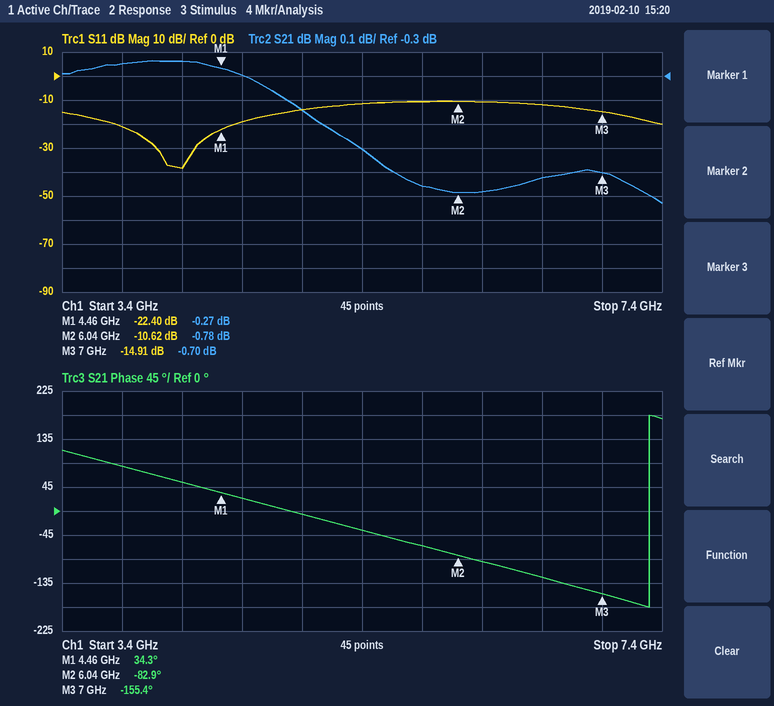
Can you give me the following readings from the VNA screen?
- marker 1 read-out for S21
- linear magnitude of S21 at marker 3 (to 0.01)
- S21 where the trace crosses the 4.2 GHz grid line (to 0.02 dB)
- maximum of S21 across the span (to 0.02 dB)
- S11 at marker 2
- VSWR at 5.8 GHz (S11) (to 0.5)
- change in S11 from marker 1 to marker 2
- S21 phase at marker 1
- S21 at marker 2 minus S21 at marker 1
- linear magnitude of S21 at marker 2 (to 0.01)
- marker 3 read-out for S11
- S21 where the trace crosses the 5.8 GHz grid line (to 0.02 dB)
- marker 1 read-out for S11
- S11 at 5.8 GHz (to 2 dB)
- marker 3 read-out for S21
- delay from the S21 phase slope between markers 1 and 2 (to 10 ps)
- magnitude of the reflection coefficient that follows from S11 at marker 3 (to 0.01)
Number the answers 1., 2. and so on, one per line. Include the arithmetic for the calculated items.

1. -0.27 dB
2. 10^(-0.7/20) ≈ 0.92
3. -0.24 dB
4. -0.24 dB
5. -10.62 dB
6. |Γ| = 10^(-10/20) = 0.3162; VSWR = (1 + 0.3162)/(1 − 0.3162) ≈ 1.92, so 2.0 to the nearest 0.5
7. -10.62 − (-22.4) = 11.78 dB
8. 34.3°
9. -0.78 − (-0.27) = -0.51 dB
10. 10^(-0.78/20) ≈ 0.91
11. -14.91 dB
12. -0.76 dB
13. -22.40 dB
14. -10 dB
15. -0.70 dB
16. −(-82.9° − (34.3°))/(360° × 1.58 GHz) ≈ 206 ps, so 210 ps to the nearest 10 ps
17. 10^(-14.91/20) ≈ 0.18
